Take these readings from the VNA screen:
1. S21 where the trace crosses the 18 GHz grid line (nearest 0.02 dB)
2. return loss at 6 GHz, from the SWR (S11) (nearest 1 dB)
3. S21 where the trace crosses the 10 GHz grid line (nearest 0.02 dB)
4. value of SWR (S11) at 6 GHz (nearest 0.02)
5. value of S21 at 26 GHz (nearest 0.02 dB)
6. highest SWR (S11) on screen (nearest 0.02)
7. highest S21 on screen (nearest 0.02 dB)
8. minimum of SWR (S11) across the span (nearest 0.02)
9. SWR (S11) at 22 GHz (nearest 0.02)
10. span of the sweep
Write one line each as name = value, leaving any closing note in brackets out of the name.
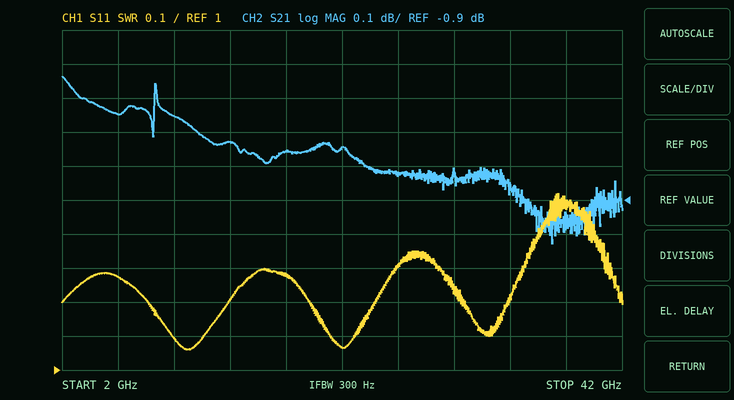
S21 where the trace crosses the 18 GHz grid line = -0.76 dB
return loss at 6 GHz, from the SWR (S11) = 18 dB
S21 where the trace crosses the 10 GHz grid line = -0.66 dB
value of SWR (S11) at 6 GHz = 1.28
value of S21 at 26 GHz = -0.82 dB
highest SWR (S11) on screen = 1.52
highest S21 on screen = -0.54 dB
minimum of SWR (S11) across the span = 1.06
SWR (S11) at 22 GHz = 1.06
span of the sweep = 40 GHz
